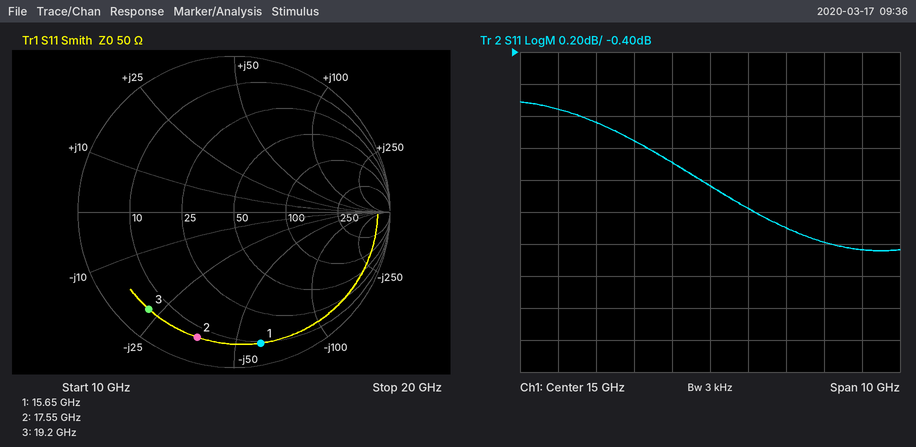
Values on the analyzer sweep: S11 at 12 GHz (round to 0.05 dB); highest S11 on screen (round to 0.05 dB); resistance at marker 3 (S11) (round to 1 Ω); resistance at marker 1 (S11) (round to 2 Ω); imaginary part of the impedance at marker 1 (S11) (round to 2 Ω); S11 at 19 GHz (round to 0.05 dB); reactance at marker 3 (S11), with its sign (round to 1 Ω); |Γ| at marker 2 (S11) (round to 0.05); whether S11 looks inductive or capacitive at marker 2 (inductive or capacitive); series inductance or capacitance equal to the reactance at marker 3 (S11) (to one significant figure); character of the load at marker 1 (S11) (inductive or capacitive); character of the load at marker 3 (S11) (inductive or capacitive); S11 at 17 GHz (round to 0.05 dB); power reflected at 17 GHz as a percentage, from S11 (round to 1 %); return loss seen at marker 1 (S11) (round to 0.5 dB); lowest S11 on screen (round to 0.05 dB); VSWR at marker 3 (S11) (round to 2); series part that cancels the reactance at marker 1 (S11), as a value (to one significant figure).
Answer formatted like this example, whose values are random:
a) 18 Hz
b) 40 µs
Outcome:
a) -0.85 dB
b) -0.70 dB
c) 6 Ω
d) 10 Ω
e) -60 Ω
f) -1.65 dB
g) -22 Ω
h) 0.85
i) capacitive
j) 400 fF
k) capacitive
l) capacitive
m) -1.50 dB
n) 71 %
o) 1.5 dB
p) -1.65 dB
q) 10
r) 600 pH
